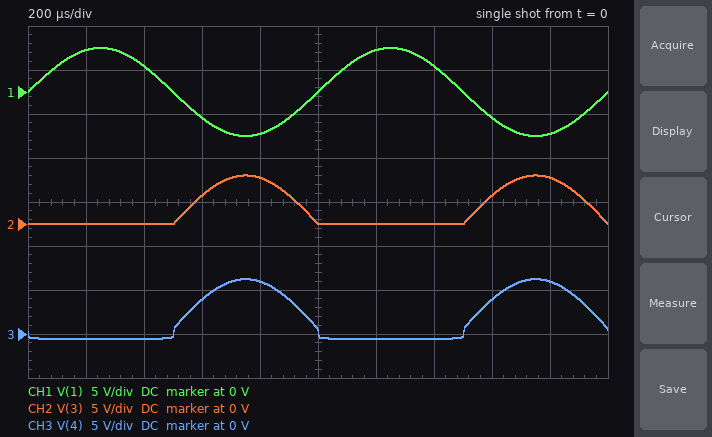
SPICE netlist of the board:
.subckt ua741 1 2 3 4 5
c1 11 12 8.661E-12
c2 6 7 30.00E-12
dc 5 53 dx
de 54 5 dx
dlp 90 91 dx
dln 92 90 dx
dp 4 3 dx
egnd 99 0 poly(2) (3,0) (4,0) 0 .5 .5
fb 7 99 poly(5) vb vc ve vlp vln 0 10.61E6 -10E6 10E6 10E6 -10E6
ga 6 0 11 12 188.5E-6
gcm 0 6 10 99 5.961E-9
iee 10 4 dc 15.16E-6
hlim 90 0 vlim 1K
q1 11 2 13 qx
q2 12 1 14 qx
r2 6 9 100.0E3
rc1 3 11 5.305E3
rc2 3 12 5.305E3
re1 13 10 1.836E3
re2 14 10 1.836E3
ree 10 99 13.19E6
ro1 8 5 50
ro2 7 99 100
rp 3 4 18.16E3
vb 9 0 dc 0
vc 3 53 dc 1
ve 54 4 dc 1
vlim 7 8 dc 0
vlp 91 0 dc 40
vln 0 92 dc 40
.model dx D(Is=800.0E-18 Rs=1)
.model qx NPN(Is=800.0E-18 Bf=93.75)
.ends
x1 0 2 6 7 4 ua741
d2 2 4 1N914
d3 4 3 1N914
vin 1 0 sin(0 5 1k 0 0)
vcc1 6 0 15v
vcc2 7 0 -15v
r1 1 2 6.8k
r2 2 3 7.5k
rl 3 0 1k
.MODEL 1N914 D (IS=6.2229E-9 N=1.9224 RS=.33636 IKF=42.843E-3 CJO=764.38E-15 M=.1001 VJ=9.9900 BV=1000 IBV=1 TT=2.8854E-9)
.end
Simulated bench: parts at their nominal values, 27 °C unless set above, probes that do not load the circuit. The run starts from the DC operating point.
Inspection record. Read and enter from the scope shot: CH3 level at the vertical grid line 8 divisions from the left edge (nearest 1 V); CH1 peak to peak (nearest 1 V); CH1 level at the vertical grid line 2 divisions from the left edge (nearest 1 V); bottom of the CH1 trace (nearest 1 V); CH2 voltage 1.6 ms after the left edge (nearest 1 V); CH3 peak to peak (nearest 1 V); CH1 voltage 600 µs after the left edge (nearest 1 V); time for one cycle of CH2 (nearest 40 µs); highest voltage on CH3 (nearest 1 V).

4 V
10 V
3 V
-5 V
3 V
7 V
-3 V
1.00 ms
6 V
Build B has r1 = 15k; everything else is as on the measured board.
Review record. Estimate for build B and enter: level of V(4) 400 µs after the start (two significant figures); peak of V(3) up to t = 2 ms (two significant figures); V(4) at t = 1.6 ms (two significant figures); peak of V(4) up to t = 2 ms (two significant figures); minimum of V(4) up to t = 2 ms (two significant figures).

-520 mV
2.5 V
2.1 V
3.2 V
-550 mV
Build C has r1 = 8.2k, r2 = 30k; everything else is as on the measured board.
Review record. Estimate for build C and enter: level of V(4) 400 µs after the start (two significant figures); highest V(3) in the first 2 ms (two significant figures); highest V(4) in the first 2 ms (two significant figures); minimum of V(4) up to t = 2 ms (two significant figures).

-550 mV
14 V
15 V
-580 mV
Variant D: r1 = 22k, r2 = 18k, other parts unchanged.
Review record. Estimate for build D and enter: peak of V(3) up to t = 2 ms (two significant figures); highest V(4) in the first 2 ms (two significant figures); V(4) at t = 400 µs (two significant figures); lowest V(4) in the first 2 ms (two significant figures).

4.1 V
4.8 V
-500 mV
-530 mV
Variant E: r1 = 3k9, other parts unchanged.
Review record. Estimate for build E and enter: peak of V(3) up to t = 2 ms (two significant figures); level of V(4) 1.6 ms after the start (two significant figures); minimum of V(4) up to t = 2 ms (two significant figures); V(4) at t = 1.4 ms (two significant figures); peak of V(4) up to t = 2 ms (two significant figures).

9.6 V
6.3 V
-620 mV
-590 mV
10 V
